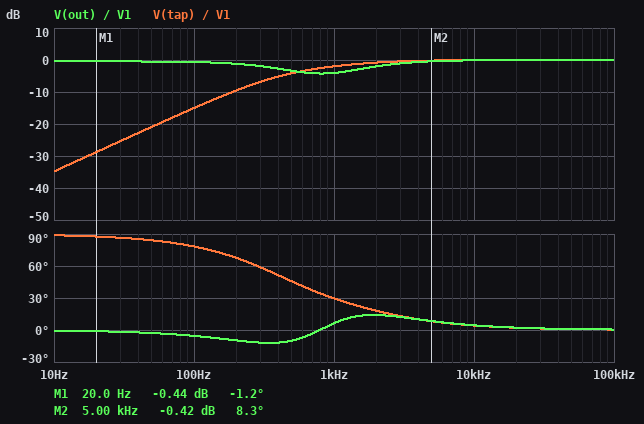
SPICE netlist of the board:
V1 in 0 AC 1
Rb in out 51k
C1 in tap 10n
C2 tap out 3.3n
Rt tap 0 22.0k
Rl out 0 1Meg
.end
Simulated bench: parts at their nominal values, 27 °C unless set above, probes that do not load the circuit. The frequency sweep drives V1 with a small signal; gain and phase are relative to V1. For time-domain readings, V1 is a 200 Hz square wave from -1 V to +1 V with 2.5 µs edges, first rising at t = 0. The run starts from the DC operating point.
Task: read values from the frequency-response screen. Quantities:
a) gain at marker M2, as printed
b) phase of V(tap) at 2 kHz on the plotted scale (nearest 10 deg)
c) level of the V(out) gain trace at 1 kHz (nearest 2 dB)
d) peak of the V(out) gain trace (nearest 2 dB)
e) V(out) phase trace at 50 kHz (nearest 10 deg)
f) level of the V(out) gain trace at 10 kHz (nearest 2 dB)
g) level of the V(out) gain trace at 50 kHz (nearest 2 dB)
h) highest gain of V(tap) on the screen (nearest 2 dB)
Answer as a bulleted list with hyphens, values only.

- -0.42 dB
- 20 deg
- -4 dB
- 0 dB
- 0 deg
- 0 dB
- 0 dB
- 0 dB
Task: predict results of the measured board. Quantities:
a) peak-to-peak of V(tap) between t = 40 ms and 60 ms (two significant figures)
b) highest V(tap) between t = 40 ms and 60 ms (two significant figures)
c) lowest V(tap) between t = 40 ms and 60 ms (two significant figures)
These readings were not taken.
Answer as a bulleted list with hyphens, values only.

- 4.0 V
- 2.0 V
- -2.0 V
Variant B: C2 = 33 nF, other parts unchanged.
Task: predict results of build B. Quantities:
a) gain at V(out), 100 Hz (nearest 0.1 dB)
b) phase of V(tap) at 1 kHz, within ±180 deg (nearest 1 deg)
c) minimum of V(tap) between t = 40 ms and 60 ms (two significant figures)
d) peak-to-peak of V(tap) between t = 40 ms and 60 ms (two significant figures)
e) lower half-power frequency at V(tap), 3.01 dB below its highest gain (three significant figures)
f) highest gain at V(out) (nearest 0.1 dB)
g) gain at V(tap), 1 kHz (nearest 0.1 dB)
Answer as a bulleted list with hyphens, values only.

- -5.3 dB
- 29 deg
- -1.8 V
- 3.6 V
- 921 Hz
- 0 dB
- -2.7 dB
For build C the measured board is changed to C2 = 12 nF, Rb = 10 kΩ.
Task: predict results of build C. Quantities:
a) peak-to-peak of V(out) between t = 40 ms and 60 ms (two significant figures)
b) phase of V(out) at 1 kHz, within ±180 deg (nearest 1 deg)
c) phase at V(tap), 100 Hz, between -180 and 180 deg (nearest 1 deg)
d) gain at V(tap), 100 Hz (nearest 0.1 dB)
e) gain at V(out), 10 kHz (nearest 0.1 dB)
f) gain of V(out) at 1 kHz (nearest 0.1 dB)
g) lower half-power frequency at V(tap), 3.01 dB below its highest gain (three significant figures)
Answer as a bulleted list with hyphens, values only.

- 2.0 V
- 0 deg
- 71 deg
- -10.9 dB
- -0.2 dB
- -2.0 dB
- 402 Hz
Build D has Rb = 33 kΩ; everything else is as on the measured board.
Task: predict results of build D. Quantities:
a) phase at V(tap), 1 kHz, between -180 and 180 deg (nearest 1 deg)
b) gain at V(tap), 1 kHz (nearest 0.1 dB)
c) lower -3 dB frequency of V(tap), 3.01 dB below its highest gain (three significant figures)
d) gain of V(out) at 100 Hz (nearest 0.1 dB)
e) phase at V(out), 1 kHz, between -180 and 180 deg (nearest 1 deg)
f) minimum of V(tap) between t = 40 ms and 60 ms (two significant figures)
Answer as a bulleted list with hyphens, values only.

- 29 deg
- -1.8 dB
- 625 Hz
- -0.4 dB
- 0 deg
- -2.0 V
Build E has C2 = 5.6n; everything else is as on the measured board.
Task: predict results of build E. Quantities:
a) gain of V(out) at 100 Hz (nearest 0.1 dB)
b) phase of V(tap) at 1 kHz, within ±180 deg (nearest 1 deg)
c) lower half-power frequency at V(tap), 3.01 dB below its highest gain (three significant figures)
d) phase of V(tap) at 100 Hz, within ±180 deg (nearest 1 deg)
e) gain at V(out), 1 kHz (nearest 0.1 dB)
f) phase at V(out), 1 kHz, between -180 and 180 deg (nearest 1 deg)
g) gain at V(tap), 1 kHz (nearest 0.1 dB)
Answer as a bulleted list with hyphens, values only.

- -0.9 dB
- 29 deg
- 740 Hz
- 75 deg
- -4.3 dB
- 15 deg
- -2.2 dB
